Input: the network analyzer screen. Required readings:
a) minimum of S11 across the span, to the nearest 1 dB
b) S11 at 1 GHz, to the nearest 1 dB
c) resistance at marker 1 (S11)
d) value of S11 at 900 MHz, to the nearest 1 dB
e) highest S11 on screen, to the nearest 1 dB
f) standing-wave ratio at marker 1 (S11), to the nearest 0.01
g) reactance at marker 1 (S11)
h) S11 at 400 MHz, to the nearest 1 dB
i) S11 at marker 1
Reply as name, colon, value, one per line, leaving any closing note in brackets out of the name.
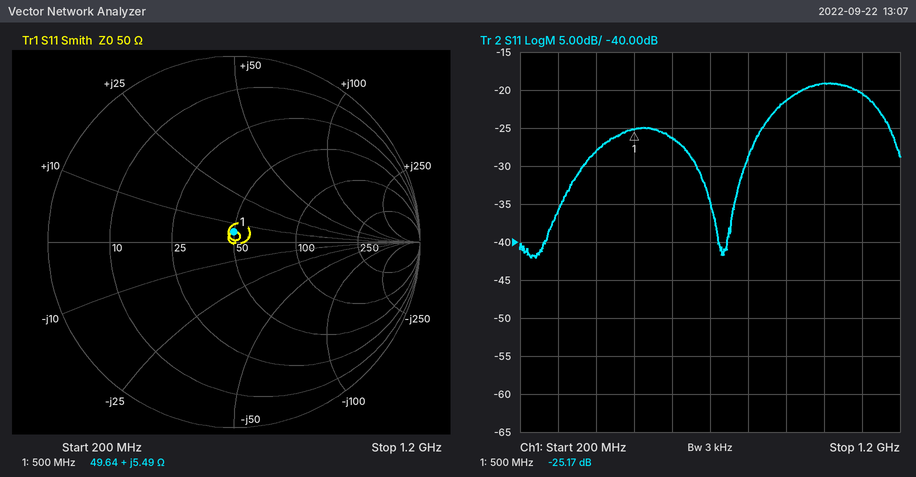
minimum of S11 across the span, to the nearest 1 dB: -42 dB
S11 at 1 GHz, to the nearest 1 dB: -19 dB
resistance at marker 1: 49.64 Ω
value of S11 at 900 MHz, to the nearest 1 dB: -21 dB
highest S11 on screen, to the nearest 1 dB: -19 dB
standing-wave ratio at marker 1 (S11), to the nearest 0.01: 1.12
reactance at marker 1: +5.49 Ω
S11 at 400 MHz, to the nearest 1 dB: -28 dB
S11 at marker 1: -25.17 dB
